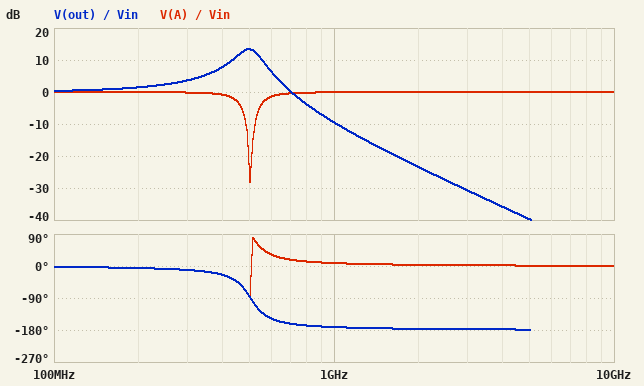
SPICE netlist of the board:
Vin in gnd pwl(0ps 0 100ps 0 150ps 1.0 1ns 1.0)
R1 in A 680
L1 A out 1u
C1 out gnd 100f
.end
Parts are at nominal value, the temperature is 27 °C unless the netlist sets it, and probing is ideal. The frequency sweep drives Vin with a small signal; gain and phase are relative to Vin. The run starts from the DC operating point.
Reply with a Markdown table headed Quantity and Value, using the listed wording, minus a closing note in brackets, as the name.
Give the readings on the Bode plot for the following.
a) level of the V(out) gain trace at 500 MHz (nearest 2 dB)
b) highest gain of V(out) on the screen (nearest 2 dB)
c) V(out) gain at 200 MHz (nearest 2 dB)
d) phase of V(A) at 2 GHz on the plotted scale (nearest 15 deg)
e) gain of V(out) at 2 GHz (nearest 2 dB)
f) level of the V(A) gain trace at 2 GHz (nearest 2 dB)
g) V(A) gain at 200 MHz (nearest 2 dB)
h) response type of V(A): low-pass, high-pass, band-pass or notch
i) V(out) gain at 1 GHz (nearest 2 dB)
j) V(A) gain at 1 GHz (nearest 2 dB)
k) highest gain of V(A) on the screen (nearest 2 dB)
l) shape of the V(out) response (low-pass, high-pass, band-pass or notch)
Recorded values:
| Quantity | Value |
|---|---|
| level of the V(out) gain trace at 500 MHz | 14 dB |
| highest gain of V(out) on the screen | 14 dB |
| V(out) gain at 200 MHz | 2 dB |
| phase of V(A) at 2 GHz on the plotted scale | 0 deg |
| gain of V(out) at 2 GHz | -24 dB |
| level of the V(A) gain trace at 2 GHz | 0 dB |
| V(A) gain at 200 MHz | 0 dB |
| response type of V(A): low-pass, high-pass, band-pass or notch | notch |
| V(out) gain at 1 GHz | -10 dB |
| V(A) gain at 1 GHz | 0 dB |
| highest gain of V(A) on the screen | 0 dB |
| shape of the V(out) response | low-pass |
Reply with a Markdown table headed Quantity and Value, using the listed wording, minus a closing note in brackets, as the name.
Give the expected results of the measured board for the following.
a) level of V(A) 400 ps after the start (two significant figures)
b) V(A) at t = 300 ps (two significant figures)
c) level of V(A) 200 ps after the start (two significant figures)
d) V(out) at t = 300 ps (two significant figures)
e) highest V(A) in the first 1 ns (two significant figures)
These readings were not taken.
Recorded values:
| Quantity | Value |
|---|---|
| level of V(A) 400 ps after the start | 850 mV |
| V(A) at t = 300 ps | 890 mV |
| level of V(A) 200 ps after the start | 950 mV |
| V(out) at t = 300 ps | 140 mV |
| highest V(A) in the first 1 ns | 980 mV |
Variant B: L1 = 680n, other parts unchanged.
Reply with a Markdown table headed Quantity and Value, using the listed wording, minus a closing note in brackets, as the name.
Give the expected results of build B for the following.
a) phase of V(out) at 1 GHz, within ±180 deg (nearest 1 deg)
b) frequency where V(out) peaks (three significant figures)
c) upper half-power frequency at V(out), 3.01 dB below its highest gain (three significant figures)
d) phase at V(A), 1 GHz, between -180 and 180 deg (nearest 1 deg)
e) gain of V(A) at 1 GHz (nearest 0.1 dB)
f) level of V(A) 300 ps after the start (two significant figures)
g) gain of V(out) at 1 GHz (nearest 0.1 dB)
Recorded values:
| Quantity | Value |
|---|---|
| phase of V(out) at 1 GHz, within ±180 deg | -166 deg |
| frequency where V(out) peaks | 600 MHz |
| upper half-power frequency at V(out), 3.01 dB below its highest gain | 675 MHz |
| phase at V(A), 1 GHz, between -180 and 180 deg | 14 deg |
| gain of V(A) at 1 GHz | -0.3 dB |
| level of V(A) 300 ps after the start | 850 mV |
| gain of V(out) at 1 GHz | -4.8 dB |
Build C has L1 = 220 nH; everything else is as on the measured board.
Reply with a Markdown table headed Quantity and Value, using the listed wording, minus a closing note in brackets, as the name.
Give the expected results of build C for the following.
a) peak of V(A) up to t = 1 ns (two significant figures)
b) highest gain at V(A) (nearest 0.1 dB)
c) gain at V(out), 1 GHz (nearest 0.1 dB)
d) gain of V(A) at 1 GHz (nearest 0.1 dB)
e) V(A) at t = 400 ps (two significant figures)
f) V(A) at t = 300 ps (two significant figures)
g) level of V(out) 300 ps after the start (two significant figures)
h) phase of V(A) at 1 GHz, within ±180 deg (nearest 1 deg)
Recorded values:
| Quantity | Value |
|---|---|
| peak of V(A) up to t = 1 ns | 1.2 V |
| highest gain at V(A) | 0 dB |
| gain at V(out), 1 GHz | 7.0 dB |
| gain of V(A) at 1 GHz | -10.6 dB |
| V(A) at t = 400 ps | 700 mV |
| V(A) at t = 300 ps | 670 mV |
| level of V(out) 300 ps after the start | 520 mV |
| phase of V(A) at 1 GHz, within ±180 deg | -73 deg |
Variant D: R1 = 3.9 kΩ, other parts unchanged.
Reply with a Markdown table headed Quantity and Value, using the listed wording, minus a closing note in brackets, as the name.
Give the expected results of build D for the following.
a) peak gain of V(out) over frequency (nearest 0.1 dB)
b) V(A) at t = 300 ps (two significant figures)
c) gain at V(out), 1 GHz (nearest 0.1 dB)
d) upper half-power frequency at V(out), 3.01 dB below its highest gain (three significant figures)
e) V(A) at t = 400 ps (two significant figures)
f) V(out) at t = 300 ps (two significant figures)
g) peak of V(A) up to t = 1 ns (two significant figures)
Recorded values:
| Quantity | Value |
|---|---|
| peak gain of V(out) over frequency | 0.3 dB |
| V(A) at t = 300 ps | 530 mV |
| gain at V(out), 1 GHz | -11.7 dB |
| upper half-power frequency at V(out), 3.01 dB below its highest gain | 554 MHz |
| V(A) at t = 400 ps | 420 mV |
| V(out) at t = 300 ps | 120 mV |
| peak of V(A) up to t = 1 ns | 910 mV |
